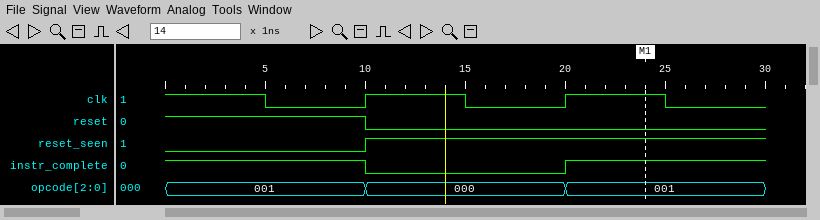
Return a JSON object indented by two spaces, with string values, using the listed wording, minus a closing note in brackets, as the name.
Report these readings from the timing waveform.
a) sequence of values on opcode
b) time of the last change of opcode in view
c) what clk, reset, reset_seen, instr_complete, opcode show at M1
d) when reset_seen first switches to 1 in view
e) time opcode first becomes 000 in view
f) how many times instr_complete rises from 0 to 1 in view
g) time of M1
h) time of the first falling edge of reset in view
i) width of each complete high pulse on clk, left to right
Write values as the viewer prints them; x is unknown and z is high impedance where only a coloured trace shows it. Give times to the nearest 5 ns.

{
  "sequence of values on opcode": "001, 000, 001",
  "time of the last change of opcode in view": "20 ns",
  "what clk, reset, reset_seen, instr_complete, opcode show at M1": "clk=1, reset=0, reset_seen=1, instr_complete=1, opcode=001",
  "when reset_seen first switches to 1 in view": "10 ns",
  "time opcode first becomes 000 in view": "10 ns",
  "how many times instr_complete rises from 0 to 1 in view": "1",
  "time of M1": "25 ns",
  "time of the first falling edge of reset in view": "10 ns",
  "width of each complete high pulse on clk, left to right": "5 ns, 5 ns"
}
